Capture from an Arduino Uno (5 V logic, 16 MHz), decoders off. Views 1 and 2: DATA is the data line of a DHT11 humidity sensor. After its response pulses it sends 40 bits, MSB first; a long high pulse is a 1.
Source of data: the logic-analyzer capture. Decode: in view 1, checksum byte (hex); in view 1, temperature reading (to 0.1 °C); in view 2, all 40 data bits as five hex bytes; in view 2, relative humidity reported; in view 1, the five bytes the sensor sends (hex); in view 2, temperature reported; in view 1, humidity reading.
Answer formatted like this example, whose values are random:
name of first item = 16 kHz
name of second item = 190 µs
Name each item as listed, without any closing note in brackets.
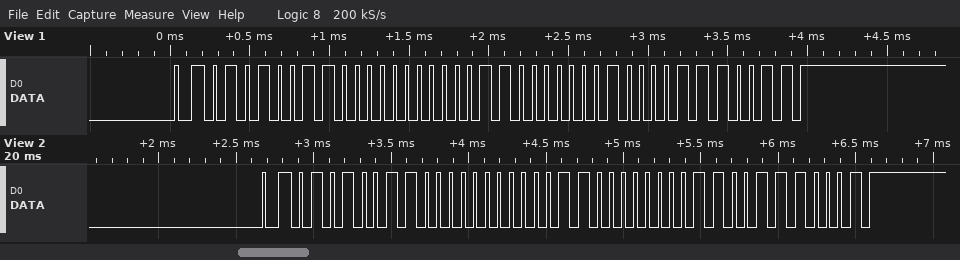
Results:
in view 1, checksum byte = 0x73
in view 1, temperature reading = 24.8 °C
in view 2, all 40 data bits as five hex bytes = 53 00 18 06 71
in view 2, relative humidity reported = 83 %
in view 1, the five bytes the sensor sends = 53 00 18 08 73
in view 2, temperature reported = 24.6 °C
in view 1, humidity reading = 83 %
